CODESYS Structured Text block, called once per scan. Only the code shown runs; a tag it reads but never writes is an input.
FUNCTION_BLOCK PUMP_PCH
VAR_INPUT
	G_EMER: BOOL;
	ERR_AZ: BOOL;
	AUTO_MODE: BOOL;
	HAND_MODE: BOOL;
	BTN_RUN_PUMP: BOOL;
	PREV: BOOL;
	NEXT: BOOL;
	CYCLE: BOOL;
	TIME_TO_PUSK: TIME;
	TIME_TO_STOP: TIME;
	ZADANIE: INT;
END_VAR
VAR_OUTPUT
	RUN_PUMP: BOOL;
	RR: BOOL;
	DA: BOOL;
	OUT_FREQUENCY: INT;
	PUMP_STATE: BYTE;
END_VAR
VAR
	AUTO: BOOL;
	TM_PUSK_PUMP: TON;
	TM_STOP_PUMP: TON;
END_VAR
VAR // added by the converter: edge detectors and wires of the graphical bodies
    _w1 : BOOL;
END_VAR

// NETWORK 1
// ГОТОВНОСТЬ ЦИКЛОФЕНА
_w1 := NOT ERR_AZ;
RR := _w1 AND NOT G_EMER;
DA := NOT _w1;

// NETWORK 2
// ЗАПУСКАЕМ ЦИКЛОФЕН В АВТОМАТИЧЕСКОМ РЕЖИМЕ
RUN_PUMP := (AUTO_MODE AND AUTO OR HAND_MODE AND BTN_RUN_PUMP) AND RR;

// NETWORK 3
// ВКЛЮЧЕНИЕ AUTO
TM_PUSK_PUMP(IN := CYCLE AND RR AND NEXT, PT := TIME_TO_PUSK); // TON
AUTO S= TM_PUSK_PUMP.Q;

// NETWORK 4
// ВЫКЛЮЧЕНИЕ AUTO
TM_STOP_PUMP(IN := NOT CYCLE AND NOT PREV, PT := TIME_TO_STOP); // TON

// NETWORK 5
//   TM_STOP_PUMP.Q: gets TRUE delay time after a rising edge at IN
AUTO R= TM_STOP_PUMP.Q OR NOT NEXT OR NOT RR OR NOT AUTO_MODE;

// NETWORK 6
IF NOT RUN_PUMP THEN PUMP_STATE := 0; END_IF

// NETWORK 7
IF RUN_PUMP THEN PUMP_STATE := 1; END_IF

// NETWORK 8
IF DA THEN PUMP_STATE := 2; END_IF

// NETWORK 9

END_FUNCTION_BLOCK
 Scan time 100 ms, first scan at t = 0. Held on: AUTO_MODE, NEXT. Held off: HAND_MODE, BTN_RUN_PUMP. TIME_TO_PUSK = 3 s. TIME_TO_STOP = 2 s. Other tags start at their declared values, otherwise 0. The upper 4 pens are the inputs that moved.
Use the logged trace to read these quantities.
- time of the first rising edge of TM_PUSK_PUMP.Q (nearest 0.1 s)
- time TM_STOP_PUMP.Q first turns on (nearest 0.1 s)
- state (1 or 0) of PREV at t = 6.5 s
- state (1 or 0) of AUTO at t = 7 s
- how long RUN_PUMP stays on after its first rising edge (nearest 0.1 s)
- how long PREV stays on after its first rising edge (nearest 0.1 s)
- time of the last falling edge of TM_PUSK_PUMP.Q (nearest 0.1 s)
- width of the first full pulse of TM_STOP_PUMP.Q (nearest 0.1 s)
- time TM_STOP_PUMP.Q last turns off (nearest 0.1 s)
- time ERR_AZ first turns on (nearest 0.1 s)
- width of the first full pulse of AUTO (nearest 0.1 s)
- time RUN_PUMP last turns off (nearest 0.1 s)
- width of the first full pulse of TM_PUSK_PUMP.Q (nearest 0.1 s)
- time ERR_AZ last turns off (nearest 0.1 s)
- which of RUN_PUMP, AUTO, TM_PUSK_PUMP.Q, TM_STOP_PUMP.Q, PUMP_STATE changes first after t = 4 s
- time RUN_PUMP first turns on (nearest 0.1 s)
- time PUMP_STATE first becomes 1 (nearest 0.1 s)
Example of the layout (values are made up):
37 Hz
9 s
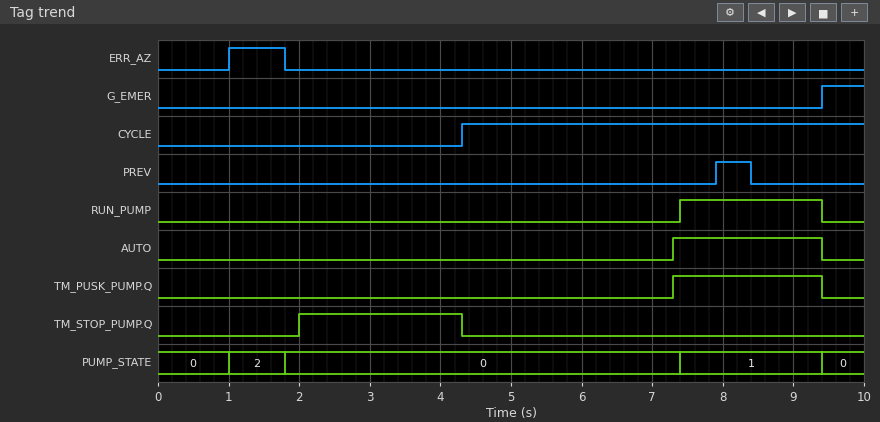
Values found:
7.3 s
2.0 s
0
0
2.0 s
0.5 s
9.4 s
2.3 s
4.3 s
1.0 s
2.1 s
9.4 s
2.1 s
1.8 s
TM_STOP_PUMP.Q
7.4 s
7.4 s
